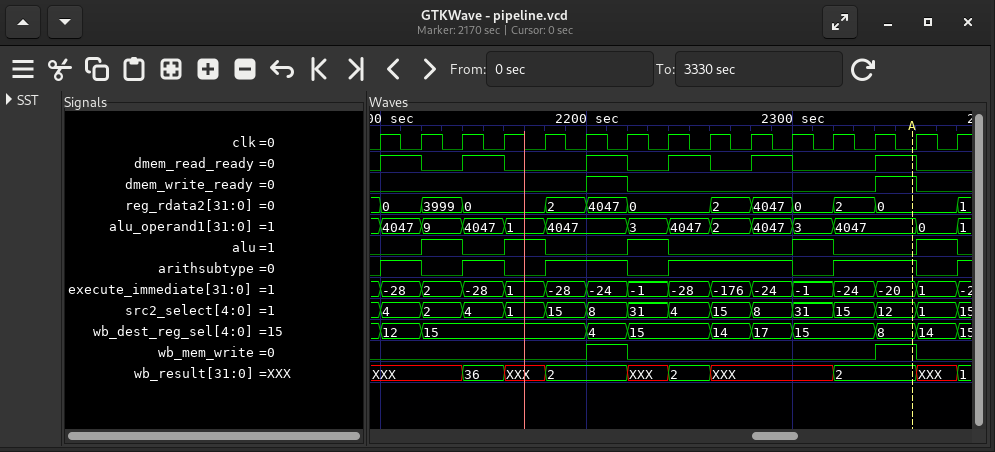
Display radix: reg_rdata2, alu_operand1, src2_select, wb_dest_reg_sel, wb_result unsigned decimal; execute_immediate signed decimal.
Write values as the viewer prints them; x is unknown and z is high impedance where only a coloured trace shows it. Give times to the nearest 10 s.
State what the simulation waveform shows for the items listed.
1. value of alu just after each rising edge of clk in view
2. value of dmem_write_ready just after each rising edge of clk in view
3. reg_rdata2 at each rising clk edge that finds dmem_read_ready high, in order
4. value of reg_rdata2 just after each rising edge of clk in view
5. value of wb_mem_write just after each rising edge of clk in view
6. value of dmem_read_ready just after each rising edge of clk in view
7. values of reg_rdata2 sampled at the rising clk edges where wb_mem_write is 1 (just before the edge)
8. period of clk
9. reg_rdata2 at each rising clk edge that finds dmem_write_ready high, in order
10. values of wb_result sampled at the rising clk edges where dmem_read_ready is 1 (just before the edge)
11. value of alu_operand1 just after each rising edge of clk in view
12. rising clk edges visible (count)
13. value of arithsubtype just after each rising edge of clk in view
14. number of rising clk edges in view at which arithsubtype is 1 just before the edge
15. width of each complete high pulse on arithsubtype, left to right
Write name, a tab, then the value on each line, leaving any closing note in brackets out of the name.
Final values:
value of alu just after each rising edge of clk in view	0 1 0 1 0 0 1 0 0 0 1 0 0 1 0
value of dmem_write_ready just after each rising edge of clk in view	0 0 0 0 0 1 0 0 0 0 0 0 1 0 0
reg_rdata2 at each rising clk edge that finds dmem_read_ready high, in order	0, 0, 4047, 0, 4047, 0
value of reg_rdata2 just after each rising edge of clk in view	0, 3999, 0, 0, 2, 4047, 0, 0, 2, 4047, 0, 2, 0, 0, 1
value of wb_mem_write just after each rising edge of clk in view	0 0 0 0 0 1 0 0 0 0 0 0 1 0 0
value of dmem_read_ready just after each rising edge of clk in view	1 0 1 0 0 1 0 1 0 1 0 0 1 0 0
values of reg_rdata2 sampled at the rising clk edges where wb_mem_write is 1	4047, 0
period of clk	20 s
reg_rdata2 at each rising clk edge that finds dmem_write_ready high, in order	4047, 0
values of wb_result sampled at the rising clk edges where dmem_read_ready is 1	XXX, 36, 2, 2, XXX, 2
value of alu_operand1 just after each rising edge of clk in view	4047, 9, 4047, 1, 4047, 4047, 3, 4047, 2, 4047, 3, 4047, 4047, 0, 1
rising clk edges visible	15
value of arithsubtype just after each rising edge of clk in view	1 0 1 0 1 1 0 1 1 1 0 1 1 0 1
number of rising clk edges in view at which arithsubtype is 1 just before the edge	9
width of each complete high pulse on arithsubtype, left to right	20 s, 20 s, 40 s, 60 s, 40 s
